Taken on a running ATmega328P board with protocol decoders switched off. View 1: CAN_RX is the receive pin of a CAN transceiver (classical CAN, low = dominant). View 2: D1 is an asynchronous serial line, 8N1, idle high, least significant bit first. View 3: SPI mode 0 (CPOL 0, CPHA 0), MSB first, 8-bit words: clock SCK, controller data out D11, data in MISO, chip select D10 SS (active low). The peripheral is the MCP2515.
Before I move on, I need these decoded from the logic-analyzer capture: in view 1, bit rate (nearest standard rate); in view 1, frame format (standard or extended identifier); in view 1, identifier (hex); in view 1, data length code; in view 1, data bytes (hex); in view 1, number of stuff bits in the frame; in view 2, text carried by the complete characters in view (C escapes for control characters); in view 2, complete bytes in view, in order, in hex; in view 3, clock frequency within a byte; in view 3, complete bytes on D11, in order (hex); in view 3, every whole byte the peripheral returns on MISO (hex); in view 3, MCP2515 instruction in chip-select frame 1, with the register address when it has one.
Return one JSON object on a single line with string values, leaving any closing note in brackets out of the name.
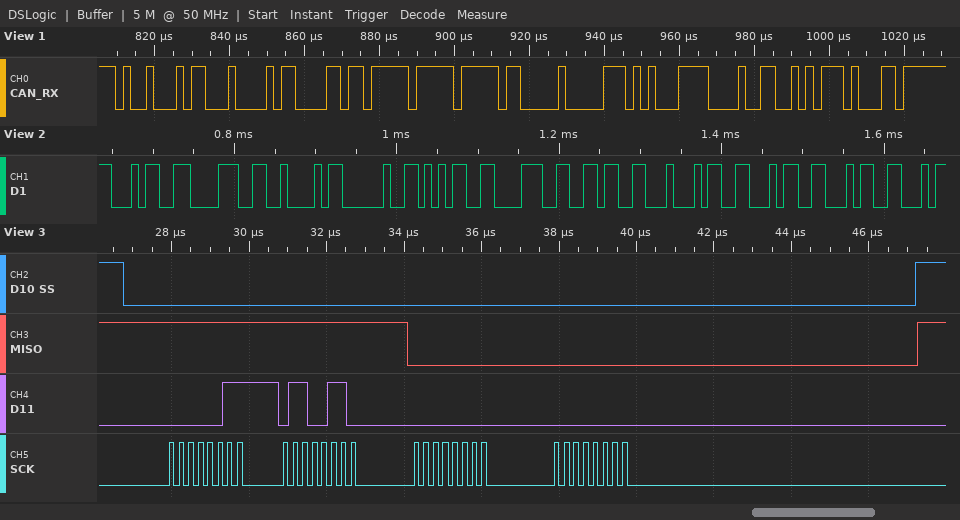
{"in view 1, bit rate": "500 kbit/s", "in view 1, frame format": "standard", "in view 1, identifier": "0x48B", "in view 1, data length code": "8", "in view 1, data bytes": "58 6D FF FF 00 35 1E 13", "in view 1, number of stuff bits in the frame": "5", "in view 2, text carried by the complete characters in view": "\"48B 586DFFF\"", "in view 2, complete bytes in view, in order, in hex": "34 38 42 20 35 38 36 44 46 46 46", "in view 3, clock frequency within a byte": "4 MHz", "in view 3, complete bytes on D11, in order": "0x03 0x66 0x00 0x00", "in view 3, every whole byte the peripheral returns on MISO": "0xFF 0xFF 0x00 0x00", "in view 3, MCP2515 instruction in chip-select frame 1, with the register address when it has one": "READ 0x66"}
